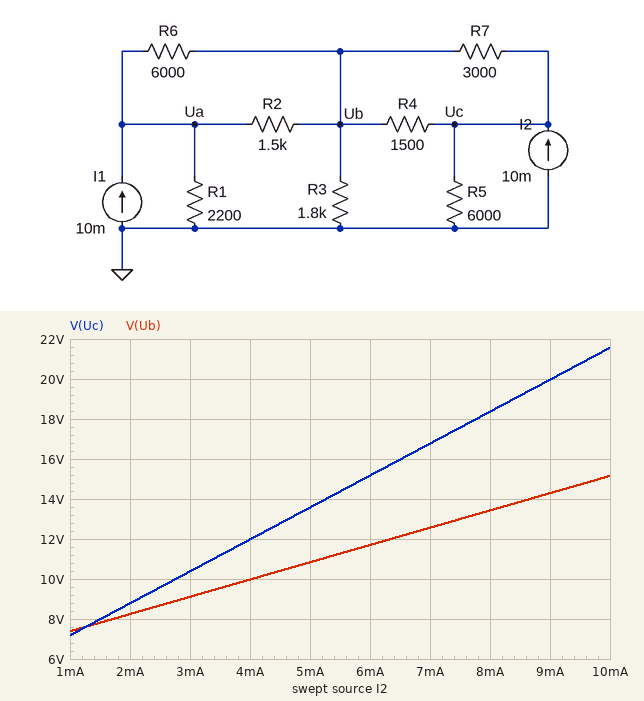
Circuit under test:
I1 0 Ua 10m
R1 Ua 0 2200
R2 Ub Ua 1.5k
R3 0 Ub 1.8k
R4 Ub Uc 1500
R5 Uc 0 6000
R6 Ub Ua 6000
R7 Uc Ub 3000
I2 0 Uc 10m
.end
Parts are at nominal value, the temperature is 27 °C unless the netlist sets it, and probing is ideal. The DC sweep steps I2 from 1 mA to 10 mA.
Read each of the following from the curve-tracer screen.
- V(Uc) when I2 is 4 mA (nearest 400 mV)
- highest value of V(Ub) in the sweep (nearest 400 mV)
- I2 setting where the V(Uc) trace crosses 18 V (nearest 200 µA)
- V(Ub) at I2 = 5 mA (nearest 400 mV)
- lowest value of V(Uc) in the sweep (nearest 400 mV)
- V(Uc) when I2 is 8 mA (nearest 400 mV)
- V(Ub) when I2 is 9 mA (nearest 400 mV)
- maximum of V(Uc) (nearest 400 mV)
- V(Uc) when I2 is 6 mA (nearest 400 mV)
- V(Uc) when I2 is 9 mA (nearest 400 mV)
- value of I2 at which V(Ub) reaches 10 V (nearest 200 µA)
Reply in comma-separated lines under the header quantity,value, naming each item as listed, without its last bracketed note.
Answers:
quantity,value
V(Uc) when I2 is 4 mA,12.0 V
highest value of V(Ub) in the sweep,15.2 V
I2 setting where the V(Uc) trace crosses 18 V,7.8 mA
V(Ub) at I2 = 5 mA,10.8 V
lowest value of V(Uc) in the sweep,7.2 V
V(Uc) when I2 is 8 mA,18.4 V
V(Ub) when I2 is 9 mA,14.4 V
maximum of V(Uc),21.6 V
V(Uc) when I2 is 6 mA,15.2 V
V(Uc) when I2 is 9 mA,20.0 V
value of I2 at which V(Ub) reaches 10 V,4.0 mA
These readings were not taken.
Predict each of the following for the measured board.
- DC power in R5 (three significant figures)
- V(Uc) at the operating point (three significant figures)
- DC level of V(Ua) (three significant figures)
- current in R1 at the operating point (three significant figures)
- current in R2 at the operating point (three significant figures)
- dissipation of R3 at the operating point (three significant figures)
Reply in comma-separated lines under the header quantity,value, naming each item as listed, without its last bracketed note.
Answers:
quantity,value
DC power in R5,77.5 mW
V(Uc) at the operating point,21.6 V
DC level of V(Ua),17.6 V
current in R1 at the operating point,7.99 mA
current in R2 at the operating point,1.61 mA
dissipation of R3 at the operating point,128 mW
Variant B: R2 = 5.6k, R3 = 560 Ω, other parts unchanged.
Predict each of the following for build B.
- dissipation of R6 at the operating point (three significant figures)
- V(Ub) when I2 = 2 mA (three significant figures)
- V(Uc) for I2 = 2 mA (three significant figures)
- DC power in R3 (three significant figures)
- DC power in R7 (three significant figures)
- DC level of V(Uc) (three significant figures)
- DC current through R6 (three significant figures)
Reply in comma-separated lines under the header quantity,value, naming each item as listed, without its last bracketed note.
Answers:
quantity,value
dissipation of R6 at the operating point,13.7 mW
V(Ub) when I2 = 2 mA,2.84 V
V(Uc) for I2 = 2 mA,4.15 V
DC power in R3,65.7 mW
DC power in R7,19.8 mW
DC level of V(Uc),13.8 V
DC current through R6,1.51 mA
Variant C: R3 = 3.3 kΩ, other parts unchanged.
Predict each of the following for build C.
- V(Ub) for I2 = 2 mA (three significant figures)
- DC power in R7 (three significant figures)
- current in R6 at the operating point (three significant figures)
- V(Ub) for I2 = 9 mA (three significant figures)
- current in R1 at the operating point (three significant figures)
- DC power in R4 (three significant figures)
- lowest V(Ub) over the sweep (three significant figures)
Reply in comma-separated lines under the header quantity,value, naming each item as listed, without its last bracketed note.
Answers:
quantity,value
V(Ub) for I2 = 2 mA,11.1 V
DC power in R7,10.7 mW
current in R6 at the operating point,98.4 µA
V(Ub) for I2 = 9 mA,19.2 V
current in R1 at the operating point,9.51 mA
DC power in R4,21.4 mW
lowest V(Ub) over the sweep,9.90 V
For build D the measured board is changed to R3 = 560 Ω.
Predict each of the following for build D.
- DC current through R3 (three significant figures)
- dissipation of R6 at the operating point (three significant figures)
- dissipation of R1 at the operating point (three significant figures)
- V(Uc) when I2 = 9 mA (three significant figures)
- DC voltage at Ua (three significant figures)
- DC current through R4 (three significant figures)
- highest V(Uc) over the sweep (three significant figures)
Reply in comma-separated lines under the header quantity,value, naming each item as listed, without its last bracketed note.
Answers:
quantity,value
DC current through R3,12.1 mA
dissipation of R6 at the operating point,4.82 mW
dissipation of R1 at the operating point,67.0 mW
V(Uc) when I2 = 9 mA,13.2 V
DC voltage at Ua,12.1 V
DC current through R4,5.07 mA
highest V(Uc) over the sweep,14.4 V
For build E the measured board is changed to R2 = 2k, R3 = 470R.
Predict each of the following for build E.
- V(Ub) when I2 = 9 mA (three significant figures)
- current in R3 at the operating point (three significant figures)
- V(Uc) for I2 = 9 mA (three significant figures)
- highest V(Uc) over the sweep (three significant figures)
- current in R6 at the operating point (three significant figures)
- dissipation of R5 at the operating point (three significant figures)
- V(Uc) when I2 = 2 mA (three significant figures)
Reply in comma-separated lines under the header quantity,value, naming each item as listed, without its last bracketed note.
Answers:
quantity,value
V(Ub) when I2 = 9 mA,5.38 V
current in R3 at the operating point,12.2 mA
V(Uc) for I2 = 9 mA,12.3 V
highest V(Uc) over the sweep,13.5 V
current in R6 at the operating point,1.10 mA
dissipation of R5 at the operating point,30.2 mW
V(Uc) when I2 = 2 mA,4.30 V
